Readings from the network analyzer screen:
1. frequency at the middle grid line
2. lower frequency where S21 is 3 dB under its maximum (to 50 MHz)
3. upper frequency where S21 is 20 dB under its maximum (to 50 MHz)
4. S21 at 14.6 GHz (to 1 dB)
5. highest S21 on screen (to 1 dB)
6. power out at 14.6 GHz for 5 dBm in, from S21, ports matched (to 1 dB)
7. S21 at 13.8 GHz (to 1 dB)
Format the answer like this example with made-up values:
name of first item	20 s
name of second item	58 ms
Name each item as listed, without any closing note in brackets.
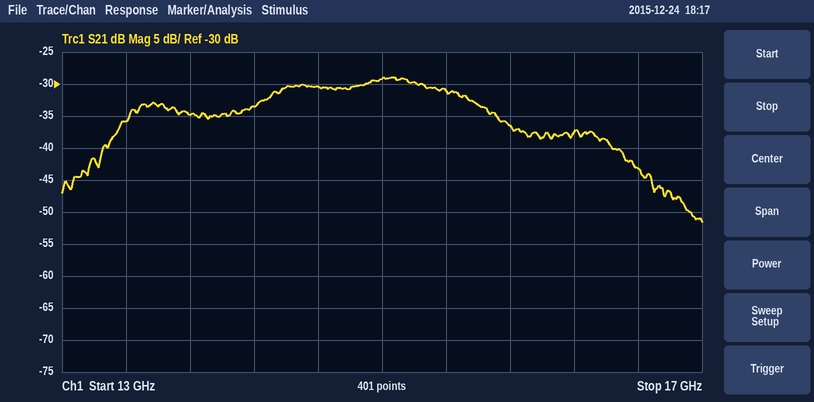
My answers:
frequency at the middle grid line	15 GHz
lower frequency where S21 is 3 dB under its maximum	14.30 GHz
upper frequency where S21 is 20 dB under its maximum	16.90 GHz
S21 at 14.6 GHz	-30 dB
highest S21 on screen	-29 dB
power out at 14.6 GHz for 5 dBm in, from S21, ports matched	-25 dBm
S21 at 13.8 GHz	-35 dB
